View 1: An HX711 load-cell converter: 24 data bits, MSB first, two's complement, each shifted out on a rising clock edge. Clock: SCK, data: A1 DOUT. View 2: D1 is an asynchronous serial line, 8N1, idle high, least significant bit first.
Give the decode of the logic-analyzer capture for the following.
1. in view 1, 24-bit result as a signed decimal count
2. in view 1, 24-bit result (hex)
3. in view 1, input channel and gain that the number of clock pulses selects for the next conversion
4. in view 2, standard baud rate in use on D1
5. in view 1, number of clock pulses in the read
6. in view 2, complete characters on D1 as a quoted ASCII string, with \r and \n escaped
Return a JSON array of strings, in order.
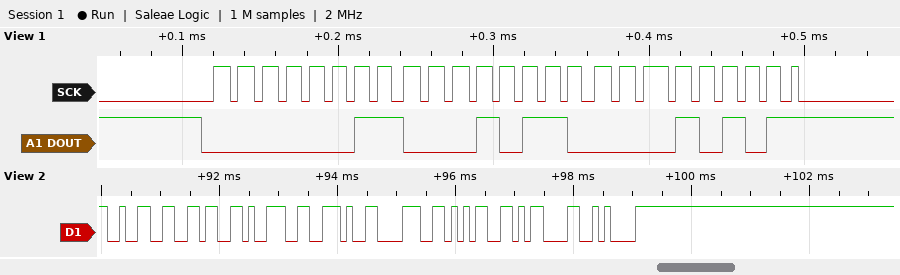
["202261", "0x031615", "channel A, gain 128", "9600 baud", "25", "\"269.85\\r\\n\""]
